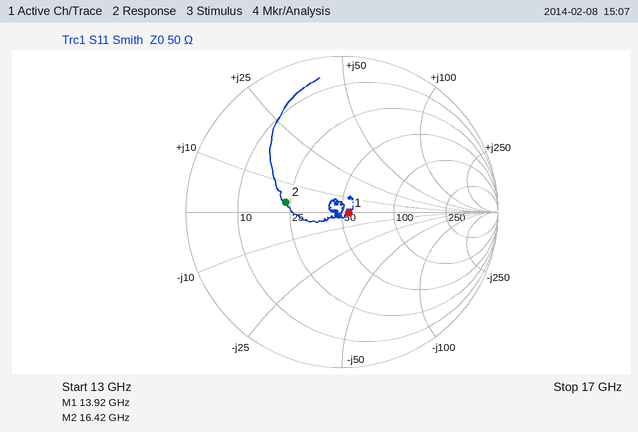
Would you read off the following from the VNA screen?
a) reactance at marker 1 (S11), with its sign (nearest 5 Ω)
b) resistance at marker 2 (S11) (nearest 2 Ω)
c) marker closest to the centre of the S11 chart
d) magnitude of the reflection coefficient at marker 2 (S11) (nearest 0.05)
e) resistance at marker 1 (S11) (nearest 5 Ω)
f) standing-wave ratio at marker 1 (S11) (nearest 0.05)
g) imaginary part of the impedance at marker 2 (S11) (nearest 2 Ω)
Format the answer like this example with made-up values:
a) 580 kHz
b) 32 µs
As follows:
a) 0 Ω
b) 24 Ω
c) marker 1
d) 0.35
e) 55 Ω
f) 1.10
g) +4 Ω
